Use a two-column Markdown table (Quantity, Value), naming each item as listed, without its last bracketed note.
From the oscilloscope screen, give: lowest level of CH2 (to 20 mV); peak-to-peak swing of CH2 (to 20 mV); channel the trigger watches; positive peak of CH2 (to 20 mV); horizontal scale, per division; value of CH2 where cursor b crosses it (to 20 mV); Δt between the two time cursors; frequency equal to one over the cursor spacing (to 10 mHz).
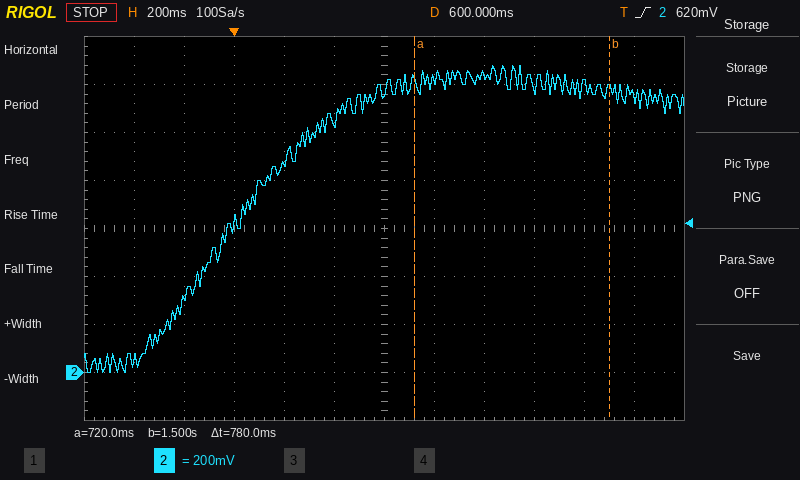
| Quantity | Value |
|---|---|
| lowest level of CH2 | 0 mV |
| peak-to-peak swing of CH2 | 1.28 V |
| channel the trigger watches | CH2 |
| positive peak of CH2 | 1.28 V |
| horizontal scale, per division | 200 ms |
| value of CH2 where cursor b crosses it | 1.18 V |
| Δt between the two time cursors | 780 ms |
| frequency equal to one over the cursor spacing | 1.28 Hz |
